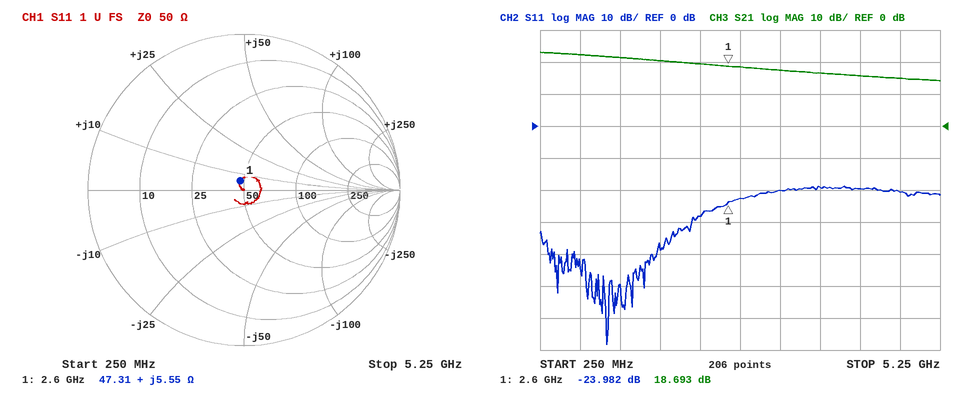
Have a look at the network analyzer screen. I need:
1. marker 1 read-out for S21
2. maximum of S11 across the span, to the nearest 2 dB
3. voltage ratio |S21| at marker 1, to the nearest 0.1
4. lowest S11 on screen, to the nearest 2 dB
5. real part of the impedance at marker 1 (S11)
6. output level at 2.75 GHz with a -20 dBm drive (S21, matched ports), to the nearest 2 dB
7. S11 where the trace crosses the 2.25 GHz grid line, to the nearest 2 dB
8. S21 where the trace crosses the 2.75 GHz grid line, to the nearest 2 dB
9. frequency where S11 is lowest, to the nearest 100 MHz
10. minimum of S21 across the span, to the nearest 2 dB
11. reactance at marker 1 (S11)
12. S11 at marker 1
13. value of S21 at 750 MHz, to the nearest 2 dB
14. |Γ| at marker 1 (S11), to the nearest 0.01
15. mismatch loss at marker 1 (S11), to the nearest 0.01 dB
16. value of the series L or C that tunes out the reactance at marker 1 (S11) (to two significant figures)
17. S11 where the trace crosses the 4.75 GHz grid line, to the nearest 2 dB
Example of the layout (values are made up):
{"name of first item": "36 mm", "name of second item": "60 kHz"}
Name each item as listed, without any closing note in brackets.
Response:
{"marker 1 read-out for S21": "18.693 dB", "maximum of S11 across the span, to the nearest 2 dB": "-18 dB", "voltage ratio |S21| at marker 1, to the nearest 0.1": "8.6", "lowest S11 on screen, to the nearest 2 dB": "-68 dB", "real part of the impedance at marker 1": "47.31 Ω", "output level at 2.75 GHz with a -20 dBm drive (S21, matched ports), to the nearest 2 dB": "-2 dBm", "S11 where the trace crosses the 2.25 GHz grid line, to the nearest 2 dB": "-28 dB", "S21 where the trace crosses the 2.75 GHz grid line, to the nearest 2 dB": "18 dB", "frequency where S11 is lowest, to the nearest 100 MHz": "1.1 GHz", "minimum of S21 across the span, to the nearest 2 dB": "14 dB", "reactance at marker 1": "+5.55 Ω", "S11 at marker 1": "-23.982 dB", "value of S21 at 750 MHz, to the nearest 2 dB": "22 dB", "|Γ| at marker 1 (S11), to the nearest 0.01": "0.06", "mismatch loss at marker 1 (S11), to the nearest 0.01 dB": "0.02 dB", "value of the series L or C that tunes out the reactance at marker 1 (S11)": "11 pF", "S11 where the trace crosses the 4.75 GHz grid line, to the nearest 2 dB": "-20 dB"}
